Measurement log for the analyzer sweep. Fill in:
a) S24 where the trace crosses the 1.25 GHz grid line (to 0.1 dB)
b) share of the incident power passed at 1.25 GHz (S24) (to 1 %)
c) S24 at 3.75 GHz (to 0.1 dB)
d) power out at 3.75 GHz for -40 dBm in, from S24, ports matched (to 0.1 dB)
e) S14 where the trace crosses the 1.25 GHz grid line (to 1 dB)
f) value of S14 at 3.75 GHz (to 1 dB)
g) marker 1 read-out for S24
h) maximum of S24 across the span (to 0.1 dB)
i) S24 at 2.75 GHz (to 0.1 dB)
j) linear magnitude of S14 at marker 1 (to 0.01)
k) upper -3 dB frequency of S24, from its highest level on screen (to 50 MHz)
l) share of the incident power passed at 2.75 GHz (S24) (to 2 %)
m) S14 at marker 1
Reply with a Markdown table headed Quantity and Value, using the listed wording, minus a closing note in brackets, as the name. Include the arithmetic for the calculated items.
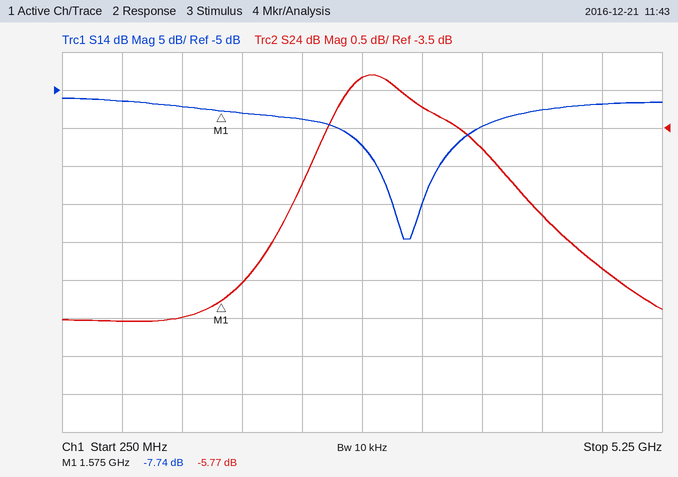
| Quantity | Value |
|---|---|
| S24 where the trace crosses the 1.25 GHz grid line | -6.0 dB |
| share of the incident power passed at 1.25 GHz (S24) | 10^(-6/10) ≈ 25 % |
| S24 at 3.75 GHz | -3.8 dB |
| power out at 3.75 GHz for -40 dBm in, from S24, ports matched | -40 dBm + (-3.8 dB) = -43.8 dBm |
| S14 where the trace crosses the 1.25 GHz grid line | -7 dB |
| value of S14 at 3.75 GHz | -10 dB |
| marker 1 read-out for S24 | -5.77 dB |
| maximum of S24 across the span | -2.8 dB |
| S24 at 2.75 GHz | -2.8 dB |
| linear magnitude of S14 at marker 1 | 10^(-7.74/20) ≈ 0.41 |
| upper -3 dB frequency of S24, from its highest level on screen | 5.15 GHz |
| share of the incident power passed at 2.75 GHz (S24) | 10^(-2.8/10) ≈ 52 % |
| S14 at marker 1 | -7.74 dB |
